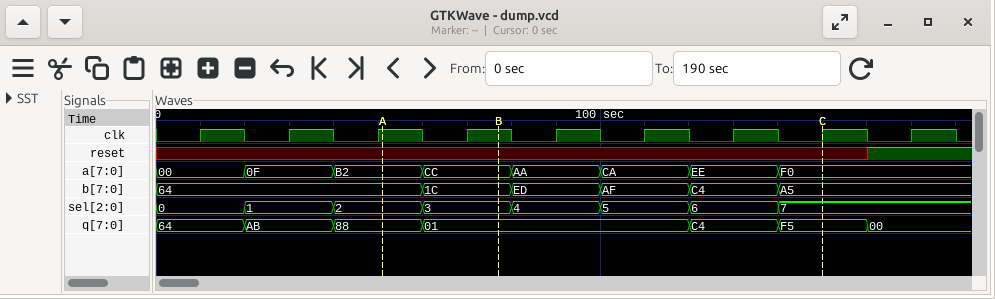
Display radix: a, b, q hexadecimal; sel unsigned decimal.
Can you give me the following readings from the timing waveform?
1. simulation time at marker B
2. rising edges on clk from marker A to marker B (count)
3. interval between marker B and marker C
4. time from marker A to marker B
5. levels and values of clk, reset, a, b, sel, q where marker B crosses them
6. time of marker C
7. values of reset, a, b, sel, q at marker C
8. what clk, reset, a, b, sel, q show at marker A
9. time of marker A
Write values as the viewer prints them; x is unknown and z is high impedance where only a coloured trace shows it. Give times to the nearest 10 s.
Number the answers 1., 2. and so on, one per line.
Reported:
1. 80 s
2. 1
3. 70 s
4. 30 s
5. clk=1, reset=x, a=CC, b=1C, sel=3, q=01
6. 150 s
7. reset=x, a=F0, b=A5, sel=7, q=F5
8. clk=1, reset=x, a=B2, b=64, sel=2, q=88
9. 50 s
